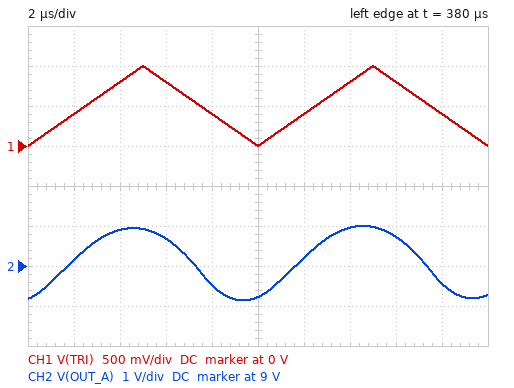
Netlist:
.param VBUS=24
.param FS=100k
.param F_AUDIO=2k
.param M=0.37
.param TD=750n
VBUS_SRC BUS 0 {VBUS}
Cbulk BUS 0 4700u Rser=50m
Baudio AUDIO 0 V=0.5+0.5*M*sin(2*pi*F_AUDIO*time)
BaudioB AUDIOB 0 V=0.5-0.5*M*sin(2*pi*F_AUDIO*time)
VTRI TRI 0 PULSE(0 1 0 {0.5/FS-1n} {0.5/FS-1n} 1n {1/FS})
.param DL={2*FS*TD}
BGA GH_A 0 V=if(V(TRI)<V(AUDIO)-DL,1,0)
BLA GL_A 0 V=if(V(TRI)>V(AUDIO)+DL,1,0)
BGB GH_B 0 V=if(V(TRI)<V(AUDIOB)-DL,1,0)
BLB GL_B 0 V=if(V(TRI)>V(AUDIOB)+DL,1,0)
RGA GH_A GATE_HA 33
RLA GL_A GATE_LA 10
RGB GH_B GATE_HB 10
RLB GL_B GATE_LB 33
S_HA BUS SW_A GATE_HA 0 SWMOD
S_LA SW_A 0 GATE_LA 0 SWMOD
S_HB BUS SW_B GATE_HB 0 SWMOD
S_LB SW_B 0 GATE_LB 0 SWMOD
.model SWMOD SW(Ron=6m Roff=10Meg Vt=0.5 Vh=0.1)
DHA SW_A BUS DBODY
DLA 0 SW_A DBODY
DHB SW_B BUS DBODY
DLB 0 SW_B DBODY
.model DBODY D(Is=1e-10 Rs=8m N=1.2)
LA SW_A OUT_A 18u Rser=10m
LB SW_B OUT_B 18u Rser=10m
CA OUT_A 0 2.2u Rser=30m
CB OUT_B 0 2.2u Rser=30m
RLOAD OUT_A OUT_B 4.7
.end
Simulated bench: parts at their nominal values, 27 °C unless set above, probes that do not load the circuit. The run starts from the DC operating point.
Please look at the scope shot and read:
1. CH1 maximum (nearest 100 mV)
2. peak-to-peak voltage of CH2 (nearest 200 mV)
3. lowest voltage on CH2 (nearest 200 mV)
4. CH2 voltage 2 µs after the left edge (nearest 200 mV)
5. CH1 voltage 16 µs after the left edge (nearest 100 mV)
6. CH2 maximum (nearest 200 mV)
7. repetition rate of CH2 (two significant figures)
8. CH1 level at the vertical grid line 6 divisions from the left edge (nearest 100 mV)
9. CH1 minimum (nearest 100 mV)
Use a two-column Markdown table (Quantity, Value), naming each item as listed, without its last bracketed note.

| Quantity | Value |
|---|---|
| CH1 maximum | 1.0 V |
| peak-to-peak voltage of CH2 | 1.8 V |
| lowest voltage on CH2 | 8.2 V |
| CH2 voltage 2 µs after the left edge | 9.2 V |
| CH1 voltage 16 µs after the left edge | 800 mV |
| CH2 maximum | 10.0 V |
| repetition rate of CH2 | 100 kHz |
| CH1 level at the vertical grid line 6 divisions from the left edge | 400 mV |
| CH1 minimum | 0 V |
